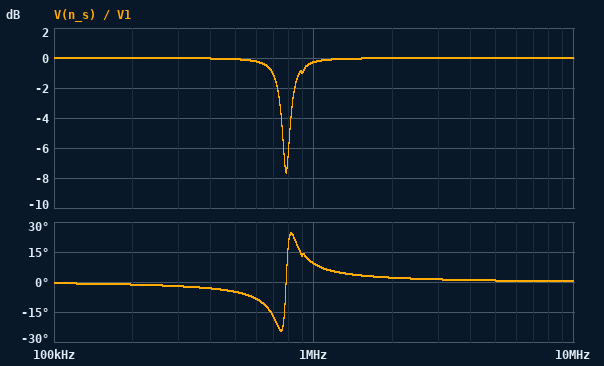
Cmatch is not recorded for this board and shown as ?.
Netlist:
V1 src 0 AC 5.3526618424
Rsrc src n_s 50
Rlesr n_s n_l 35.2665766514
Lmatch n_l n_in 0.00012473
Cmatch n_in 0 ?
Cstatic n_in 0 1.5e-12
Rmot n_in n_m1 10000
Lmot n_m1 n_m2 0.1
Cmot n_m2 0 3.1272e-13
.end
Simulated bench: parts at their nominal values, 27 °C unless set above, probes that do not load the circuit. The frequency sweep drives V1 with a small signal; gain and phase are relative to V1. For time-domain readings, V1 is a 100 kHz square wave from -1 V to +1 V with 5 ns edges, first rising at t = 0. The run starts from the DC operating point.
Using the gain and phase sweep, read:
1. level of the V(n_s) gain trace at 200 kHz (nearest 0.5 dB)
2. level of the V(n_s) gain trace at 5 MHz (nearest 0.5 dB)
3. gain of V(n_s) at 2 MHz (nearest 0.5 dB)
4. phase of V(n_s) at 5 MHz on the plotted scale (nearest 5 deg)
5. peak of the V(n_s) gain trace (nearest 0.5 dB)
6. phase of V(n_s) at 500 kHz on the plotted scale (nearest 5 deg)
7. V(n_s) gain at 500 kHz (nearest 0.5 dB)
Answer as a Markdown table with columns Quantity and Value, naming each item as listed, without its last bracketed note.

| Quantity | Value |
|---|---|
| level of the V(n_s) gain trace at 200 kHz | 0 dB |
| level of the V(n_s) gain trace at 5 MHz | 0 dB |
| gain of V(n_s) at 2 MHz | 0 dB |
| phase of V(n_s) at 5 MHz on the plotted scale | 0 deg |
| peak of the V(n_s) gain trace | 0 dB |
| phase of V(n_s) at 500 kHz on the plotted scale | -5 deg |
| V(n_s) gain at 500 kHz | 0 dB |
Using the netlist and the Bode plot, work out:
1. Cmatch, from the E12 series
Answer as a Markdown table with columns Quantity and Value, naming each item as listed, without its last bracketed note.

| Quantity | Value |
|---|---|
| Cmatch, from the E12 series | 330 pF |
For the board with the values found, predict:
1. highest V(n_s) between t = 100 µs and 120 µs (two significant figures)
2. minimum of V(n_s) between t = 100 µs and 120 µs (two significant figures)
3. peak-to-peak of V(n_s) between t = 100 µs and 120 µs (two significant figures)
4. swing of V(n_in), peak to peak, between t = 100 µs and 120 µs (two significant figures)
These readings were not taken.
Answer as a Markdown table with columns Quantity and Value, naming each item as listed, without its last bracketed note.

| Quantity | Value |
|---|---|
| highest V(n_s) between t = 100 µs and 120 µs | 1.1 V |
| minimum of V(n_s) between t = 100 µs and 120 µs | -1.1 V |
| peak-to-peak of V(n_s) between t = 100 µs and 120 µs | 2.2 V |
| swing of V(n_in), peak to peak, between t = 100 µs and 120 µs | 4.9 V |
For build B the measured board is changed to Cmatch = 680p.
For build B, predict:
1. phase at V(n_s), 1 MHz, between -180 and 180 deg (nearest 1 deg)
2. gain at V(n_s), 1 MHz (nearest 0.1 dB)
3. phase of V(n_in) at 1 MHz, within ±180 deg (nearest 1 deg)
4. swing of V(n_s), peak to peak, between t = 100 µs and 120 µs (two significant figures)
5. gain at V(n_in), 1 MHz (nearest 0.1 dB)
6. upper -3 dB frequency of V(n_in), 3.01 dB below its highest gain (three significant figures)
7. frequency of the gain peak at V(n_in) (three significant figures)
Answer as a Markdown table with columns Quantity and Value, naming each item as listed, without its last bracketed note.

| Quantity | Value |
|---|---|
| phase at V(n_s), 1 MHz, between -180 and 180 deg | 5 deg |
| gain at V(n_s), 1 MHz | -0.1 dB |
| phase of V(n_in) at 1 MHz, within ±180 deg | -171 deg |
| swing of V(n_s), peak to peak, between t = 100 µs and 120 µs | 2.3 V |
| gain at V(n_in), 1 MHz | -7.5 dB |
| upper -3 dB frequency of V(n_in), 3.01 dB below its highest gain | 592 kHz |
| frequency of the gain peak at V(n_in) | 540 kHz |
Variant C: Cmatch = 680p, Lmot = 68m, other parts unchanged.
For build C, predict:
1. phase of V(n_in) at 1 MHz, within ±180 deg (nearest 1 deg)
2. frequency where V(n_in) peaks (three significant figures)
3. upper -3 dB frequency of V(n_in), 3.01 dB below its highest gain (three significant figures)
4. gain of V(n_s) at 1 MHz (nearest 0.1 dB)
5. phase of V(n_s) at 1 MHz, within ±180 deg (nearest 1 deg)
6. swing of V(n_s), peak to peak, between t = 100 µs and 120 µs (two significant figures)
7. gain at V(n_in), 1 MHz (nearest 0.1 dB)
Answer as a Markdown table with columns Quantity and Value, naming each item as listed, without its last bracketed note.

| Quantity | Value |
|---|---|
| phase of V(n_in) at 1 MHz, within ±180 deg | -171 deg |
| frequency where V(n_in) peaks | 540 kHz |
| upper -3 dB frequency of V(n_in), 3.01 dB below its highest gain | 592 kHz |
| gain of V(n_s) at 1 MHz | -0.1 dB |
| phase of V(n_s) at 1 MHz, within ±180 deg | 5 deg |
| swing of V(n_s), peak to peak, between t = 100 µs and 120 µs | 2.3 V |
| gain at V(n_in), 1 MHz | -7.6 dB |
